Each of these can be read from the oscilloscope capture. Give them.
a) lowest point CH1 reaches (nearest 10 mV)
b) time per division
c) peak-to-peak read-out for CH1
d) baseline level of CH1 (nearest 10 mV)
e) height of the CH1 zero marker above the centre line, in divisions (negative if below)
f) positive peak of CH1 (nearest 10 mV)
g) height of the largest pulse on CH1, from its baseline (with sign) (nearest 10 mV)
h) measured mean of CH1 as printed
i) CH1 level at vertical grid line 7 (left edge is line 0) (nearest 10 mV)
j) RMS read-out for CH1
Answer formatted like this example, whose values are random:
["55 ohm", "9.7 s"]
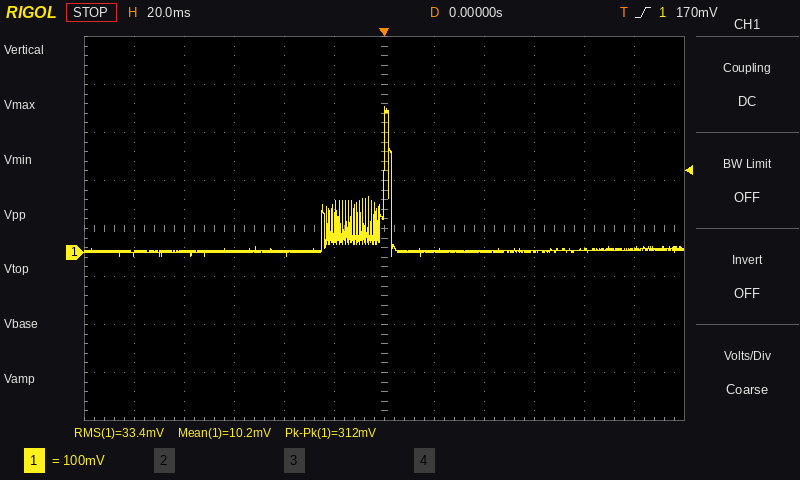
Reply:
["-10 mV", "20 ms", "312 mV", "0 mV", "-0.5 div", "300 mV", "+300 mV", "10.2 mV", "0 mV", "33.4 mV"]
